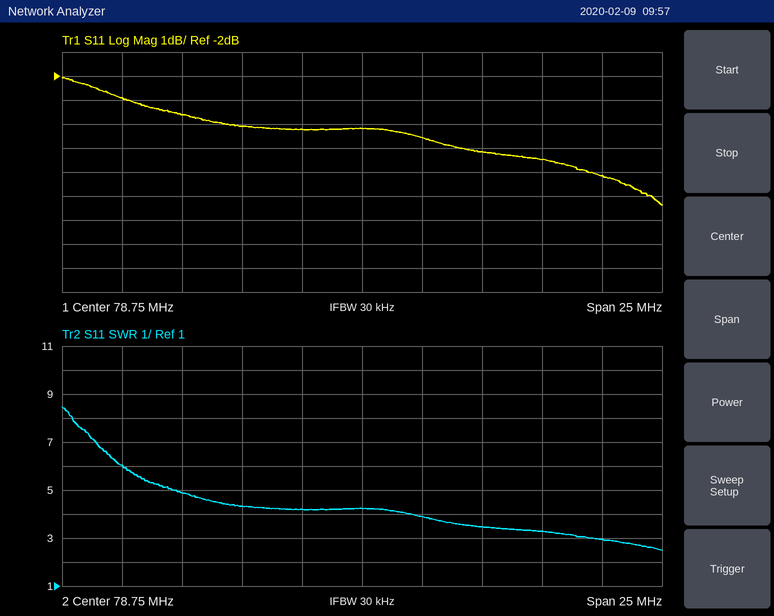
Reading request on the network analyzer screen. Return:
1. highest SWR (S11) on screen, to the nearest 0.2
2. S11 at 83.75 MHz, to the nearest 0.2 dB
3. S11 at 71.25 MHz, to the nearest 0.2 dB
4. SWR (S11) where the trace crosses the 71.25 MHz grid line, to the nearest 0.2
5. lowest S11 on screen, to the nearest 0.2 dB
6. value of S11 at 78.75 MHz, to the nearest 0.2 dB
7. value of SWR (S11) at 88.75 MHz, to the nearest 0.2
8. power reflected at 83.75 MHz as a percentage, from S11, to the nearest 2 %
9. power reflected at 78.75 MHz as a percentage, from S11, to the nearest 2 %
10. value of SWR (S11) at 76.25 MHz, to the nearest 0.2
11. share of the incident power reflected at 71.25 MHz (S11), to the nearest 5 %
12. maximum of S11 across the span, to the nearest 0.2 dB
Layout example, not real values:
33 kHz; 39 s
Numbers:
8.4; -5.2 dB; -3.6 dB; 4.8; -7.4 dB; -4.2 dB; 3.0; 30 %; 38 %; 4.2; 45 %; -2.0 dB
